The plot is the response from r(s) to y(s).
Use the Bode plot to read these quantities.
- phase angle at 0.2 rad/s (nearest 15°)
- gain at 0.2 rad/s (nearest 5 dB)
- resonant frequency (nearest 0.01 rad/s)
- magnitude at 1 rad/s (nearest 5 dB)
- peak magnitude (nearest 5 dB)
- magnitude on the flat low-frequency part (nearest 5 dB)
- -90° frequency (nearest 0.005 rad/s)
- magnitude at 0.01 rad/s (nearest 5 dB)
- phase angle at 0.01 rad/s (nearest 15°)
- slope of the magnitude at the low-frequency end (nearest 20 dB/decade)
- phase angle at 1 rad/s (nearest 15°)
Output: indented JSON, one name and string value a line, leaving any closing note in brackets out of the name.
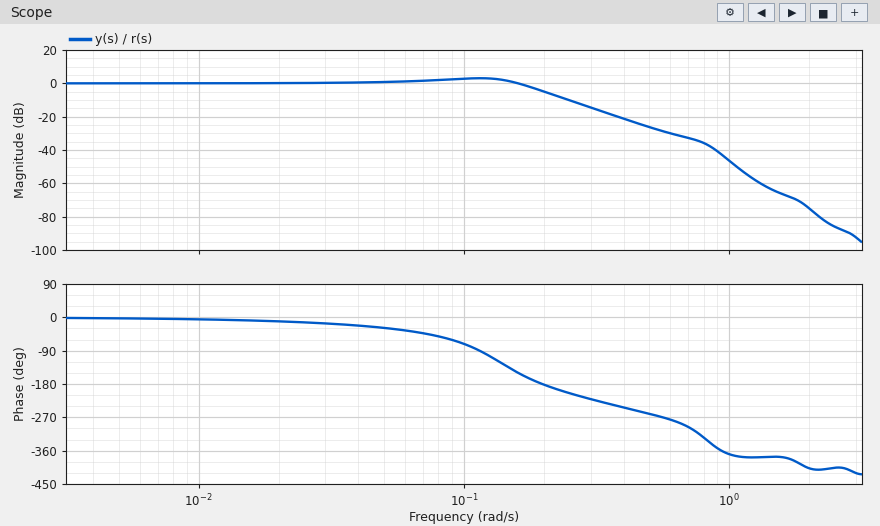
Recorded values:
{
  "phase angle at 0.2 rad/s": "-180°",
  "gain at 0.2 rad/s": "-5 dB",
  "resonant frequency": "0.11 rad/s",
  "magnitude at 1 rad/s": "-45 dB",
  "peak magnitude": "5 dB",
  "magnitude on the flat low-frequency part": "0 dB",
  "-90° frequency": "0.115 rad/s",
  "magnitude at 0.01 rad/s": "0 dB",
  "phase angle at 0.01 rad/s": "0°",
  "slope of the magnitude at the low-frequency end": "0 dB/decade",
  "phase angle at 1 rad/s": "-375°"
}
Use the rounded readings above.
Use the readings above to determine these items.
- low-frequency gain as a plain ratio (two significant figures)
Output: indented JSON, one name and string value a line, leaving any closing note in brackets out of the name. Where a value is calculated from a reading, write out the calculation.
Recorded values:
{
  "low-frequency gain as a plain ratio": "10^(0 / 20) = 1.0"
}
